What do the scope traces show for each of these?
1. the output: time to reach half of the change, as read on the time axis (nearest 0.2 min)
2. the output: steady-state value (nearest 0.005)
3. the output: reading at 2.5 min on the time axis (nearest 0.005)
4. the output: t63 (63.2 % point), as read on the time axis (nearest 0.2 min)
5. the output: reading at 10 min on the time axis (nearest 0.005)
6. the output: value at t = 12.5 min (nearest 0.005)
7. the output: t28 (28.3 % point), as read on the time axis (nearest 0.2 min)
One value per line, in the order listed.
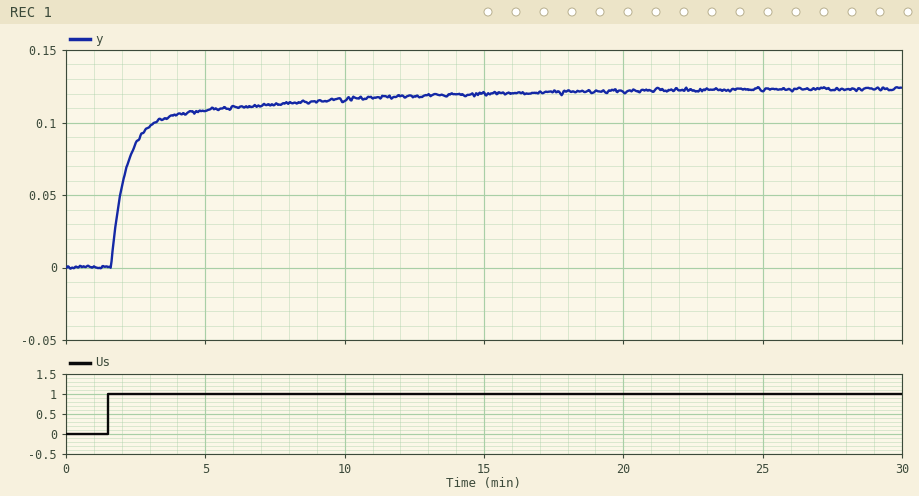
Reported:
2.0 min
0.125
0.085
2.4 min
0.115
0.120
1.8 min
